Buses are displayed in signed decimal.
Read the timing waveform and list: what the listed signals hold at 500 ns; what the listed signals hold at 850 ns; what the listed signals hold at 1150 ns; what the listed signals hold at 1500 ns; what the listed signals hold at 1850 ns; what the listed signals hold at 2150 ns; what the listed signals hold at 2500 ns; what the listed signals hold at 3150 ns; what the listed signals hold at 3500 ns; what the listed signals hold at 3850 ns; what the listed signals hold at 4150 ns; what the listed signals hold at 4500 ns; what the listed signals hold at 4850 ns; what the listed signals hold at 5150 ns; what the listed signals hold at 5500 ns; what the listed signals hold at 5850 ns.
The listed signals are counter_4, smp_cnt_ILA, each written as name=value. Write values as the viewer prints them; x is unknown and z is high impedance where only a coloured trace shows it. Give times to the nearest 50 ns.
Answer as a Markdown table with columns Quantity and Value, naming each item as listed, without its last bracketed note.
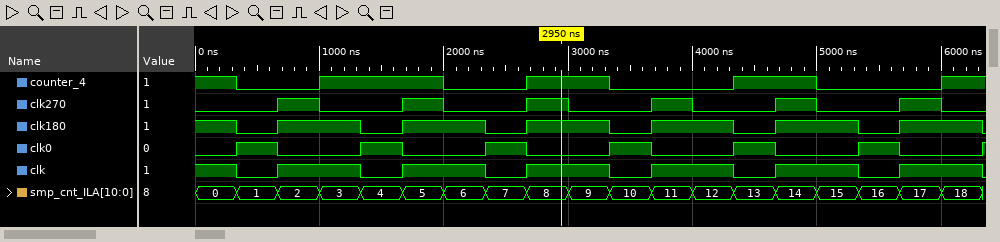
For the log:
| Quantity | Value |
|---|---|
| what the listed signals hold at 500 ns | counter_4=0, smp_cnt_ILA=1 |
| what the listed signals hold at 850 ns | counter_4=0, smp_cnt_ILA=2 |
| what the listed signals hold at 1150 ns | counter_4=1, smp_cnt_ILA=3 |
| what the listed signals hold at 1500 ns | counter_4=1, smp_cnt_ILA=4 |
| what the listed signals hold at 1850 ns | counter_4=1, smp_cnt_ILA=5 |
| what the listed signals hold at 2150 ns | counter_4=0, smp_cnt_ILA=6 |
| what the listed signals hold at 2500 ns | counter_4=0, smp_cnt_ILA=7 |
| what the listed signals hold at 3150 ns | counter_4=1, smp_cnt_ILA=9 |
| what the listed signals hold at 3500 ns | counter_4=0, smp_cnt_ILA=10 |
| what the listed signals hold at 3850 ns | counter_4=0, smp_cnt_ILA=11 |
| what the listed signals hold at 4150 ns | counter_4=0, smp_cnt_ILA=12 |
| what the listed signals hold at 4500 ns | counter_4=1, smp_cnt_ILA=13 |
| what the listed signals hold at 4850 ns | counter_4=1, smp_cnt_ILA=14 |
| what the listed signals hold at 5150 ns | counter_4=0, smp_cnt_ILA=15 |
| what the listed signals hold at 5500 ns | counter_4=0, smp_cnt_ILA=16 |
| what the listed signals hold at 5850 ns | counter_4=0, smp_cnt_ILA=17 |
